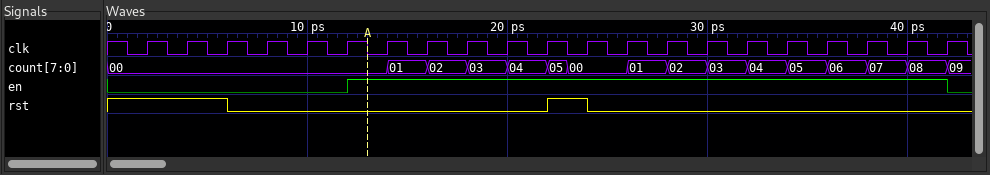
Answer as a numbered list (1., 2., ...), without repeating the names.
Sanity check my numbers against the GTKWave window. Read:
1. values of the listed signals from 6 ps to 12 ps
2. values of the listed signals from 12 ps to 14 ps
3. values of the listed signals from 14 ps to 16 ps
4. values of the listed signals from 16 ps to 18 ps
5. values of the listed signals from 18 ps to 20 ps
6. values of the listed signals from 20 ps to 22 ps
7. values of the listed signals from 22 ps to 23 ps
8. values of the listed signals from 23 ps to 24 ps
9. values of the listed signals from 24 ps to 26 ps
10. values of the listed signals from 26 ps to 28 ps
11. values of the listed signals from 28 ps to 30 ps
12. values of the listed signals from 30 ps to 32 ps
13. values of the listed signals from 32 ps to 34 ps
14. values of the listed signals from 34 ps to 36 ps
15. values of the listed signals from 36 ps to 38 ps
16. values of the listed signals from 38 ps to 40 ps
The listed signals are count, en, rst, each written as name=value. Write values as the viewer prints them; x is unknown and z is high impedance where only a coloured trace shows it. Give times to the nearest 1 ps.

1. count=00, en=0, rst=0
2. count=00, en=1, rst=0
3. count=01, en=1, rst=0
4. count=02, en=1, rst=0
5. count=03, en=1, rst=0
6. count=04, en=1, rst=0
7. count=05, en=1, rst=1
8. count=00, en=1, rst=1
9. count=00, en=1, rst=0
10. count=01, en=1, rst=0
11. count=02, en=1, rst=0
12. count=03, en=1, rst=0
13. count=04, en=1, rst=0
14. count=05, en=1, rst=0
15. count=06, en=1, rst=0
16. count=07, en=1, rst=0
